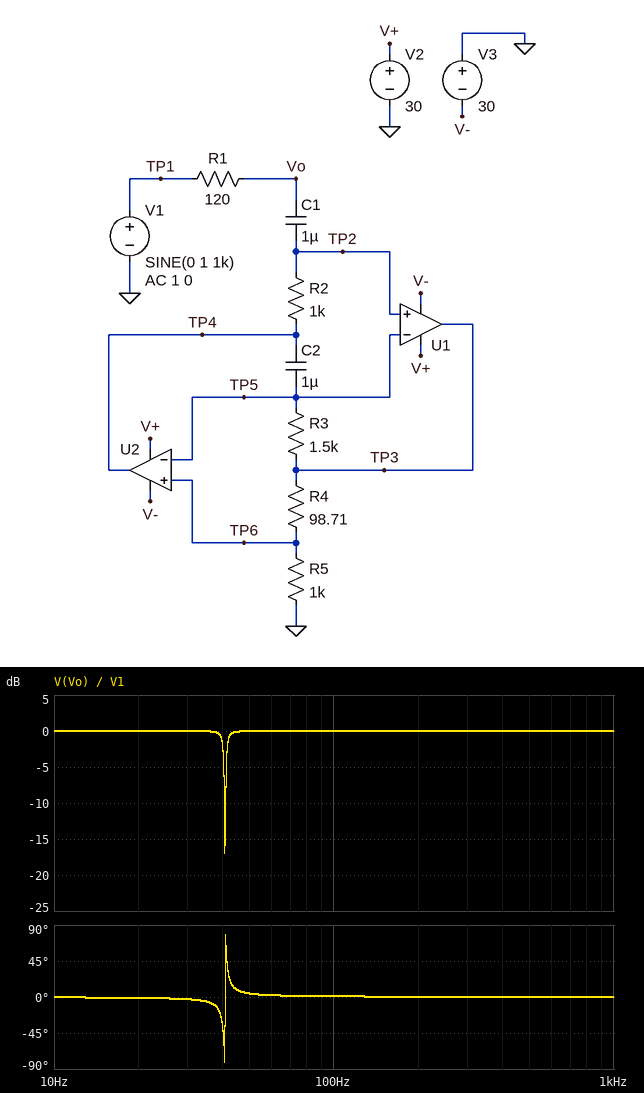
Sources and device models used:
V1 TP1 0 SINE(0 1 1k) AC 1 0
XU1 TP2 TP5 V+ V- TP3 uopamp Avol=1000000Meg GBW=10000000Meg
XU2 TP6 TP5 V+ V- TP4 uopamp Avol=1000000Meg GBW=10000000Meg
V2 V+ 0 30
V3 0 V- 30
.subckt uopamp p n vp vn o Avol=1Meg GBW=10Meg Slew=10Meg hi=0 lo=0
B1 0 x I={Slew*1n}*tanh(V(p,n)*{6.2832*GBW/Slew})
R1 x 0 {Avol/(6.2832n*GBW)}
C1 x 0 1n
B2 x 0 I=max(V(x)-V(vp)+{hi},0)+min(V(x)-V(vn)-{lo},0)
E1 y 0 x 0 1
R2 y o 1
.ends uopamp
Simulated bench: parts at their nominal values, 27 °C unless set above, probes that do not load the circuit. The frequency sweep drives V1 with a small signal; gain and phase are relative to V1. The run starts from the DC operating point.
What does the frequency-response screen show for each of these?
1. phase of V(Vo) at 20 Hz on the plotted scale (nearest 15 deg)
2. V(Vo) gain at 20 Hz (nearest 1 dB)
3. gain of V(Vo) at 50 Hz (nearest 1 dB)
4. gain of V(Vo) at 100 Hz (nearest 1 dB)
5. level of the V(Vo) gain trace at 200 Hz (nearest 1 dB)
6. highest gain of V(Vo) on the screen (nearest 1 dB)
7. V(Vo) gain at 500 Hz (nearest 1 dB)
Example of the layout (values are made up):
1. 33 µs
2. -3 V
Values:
1. 0 deg
2. 0 dB
3. 0 dB
4. 0 dB
5. 0 dB
6. 0 dB
7. 0 dB
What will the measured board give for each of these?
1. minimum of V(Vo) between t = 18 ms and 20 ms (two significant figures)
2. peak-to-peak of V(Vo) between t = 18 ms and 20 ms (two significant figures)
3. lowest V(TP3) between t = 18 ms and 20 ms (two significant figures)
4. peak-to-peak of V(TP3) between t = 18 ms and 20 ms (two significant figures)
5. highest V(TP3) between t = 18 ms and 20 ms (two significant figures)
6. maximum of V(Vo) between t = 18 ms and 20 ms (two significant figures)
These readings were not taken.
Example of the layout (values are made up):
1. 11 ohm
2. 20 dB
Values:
1. -1.0 V
2. 2.0 V
3. -1.1 V
4. 2.2 V
5. 1.1 V
6. 1.0 V
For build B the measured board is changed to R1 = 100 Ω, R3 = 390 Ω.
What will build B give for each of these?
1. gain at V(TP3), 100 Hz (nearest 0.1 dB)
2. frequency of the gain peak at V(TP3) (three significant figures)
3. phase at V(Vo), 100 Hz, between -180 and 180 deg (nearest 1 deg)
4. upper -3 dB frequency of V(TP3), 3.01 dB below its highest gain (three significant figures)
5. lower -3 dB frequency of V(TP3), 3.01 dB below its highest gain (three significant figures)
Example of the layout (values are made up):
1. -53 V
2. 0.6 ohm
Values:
1. 9.7 dB
2. 80.1 Hz
3. 6 deg
4. 82.2 Hz
5. 78.2 Hz
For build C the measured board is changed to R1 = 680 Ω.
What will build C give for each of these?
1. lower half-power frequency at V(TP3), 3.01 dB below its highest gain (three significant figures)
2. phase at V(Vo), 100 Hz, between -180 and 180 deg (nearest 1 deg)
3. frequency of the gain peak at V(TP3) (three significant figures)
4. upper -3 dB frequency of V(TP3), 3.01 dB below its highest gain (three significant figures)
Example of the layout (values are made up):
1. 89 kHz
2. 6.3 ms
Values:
1. 37.9 Hz
2. 5 deg
3. 41.1 Hz
4. 45.3 Hz
